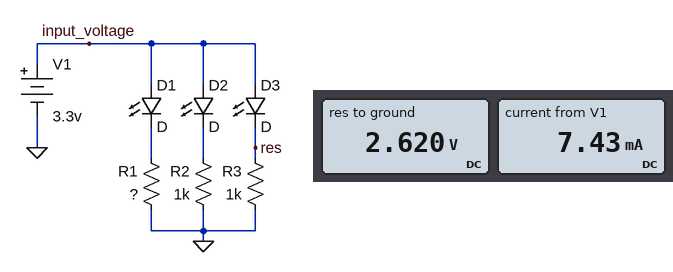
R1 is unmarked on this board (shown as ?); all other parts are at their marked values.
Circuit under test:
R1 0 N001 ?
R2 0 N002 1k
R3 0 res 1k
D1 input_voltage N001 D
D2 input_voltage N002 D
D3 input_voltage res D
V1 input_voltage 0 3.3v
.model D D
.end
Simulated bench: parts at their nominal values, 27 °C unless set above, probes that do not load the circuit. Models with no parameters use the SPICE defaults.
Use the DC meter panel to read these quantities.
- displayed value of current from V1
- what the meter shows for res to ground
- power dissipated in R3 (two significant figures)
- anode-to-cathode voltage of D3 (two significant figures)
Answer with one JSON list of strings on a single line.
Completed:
["7.43 mA", "2.620 V", "6.9 mW", "680 mV"]
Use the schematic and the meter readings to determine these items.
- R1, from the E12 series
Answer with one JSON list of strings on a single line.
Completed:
["1.2 kΩ"]
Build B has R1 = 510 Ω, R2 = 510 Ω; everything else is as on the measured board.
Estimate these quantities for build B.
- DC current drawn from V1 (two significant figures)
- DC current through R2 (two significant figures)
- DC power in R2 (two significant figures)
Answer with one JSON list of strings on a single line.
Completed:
["13 mA", "5.1 mA", "13 mW"]
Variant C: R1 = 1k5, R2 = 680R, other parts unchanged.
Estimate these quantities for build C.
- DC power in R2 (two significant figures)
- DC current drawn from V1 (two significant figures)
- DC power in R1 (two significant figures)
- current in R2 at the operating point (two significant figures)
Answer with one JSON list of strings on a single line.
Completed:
["10 mW", "8.2 mA", "4.6 mW", "3.8 mA"]
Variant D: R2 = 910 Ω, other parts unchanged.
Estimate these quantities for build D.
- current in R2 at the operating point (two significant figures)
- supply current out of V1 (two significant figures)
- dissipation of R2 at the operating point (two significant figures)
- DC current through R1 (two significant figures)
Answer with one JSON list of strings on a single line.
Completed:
["2.9 mA", "7.7 mA", "7.5 mW", "2.2 mA"]
